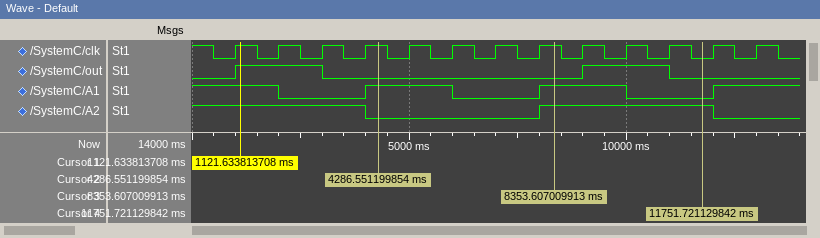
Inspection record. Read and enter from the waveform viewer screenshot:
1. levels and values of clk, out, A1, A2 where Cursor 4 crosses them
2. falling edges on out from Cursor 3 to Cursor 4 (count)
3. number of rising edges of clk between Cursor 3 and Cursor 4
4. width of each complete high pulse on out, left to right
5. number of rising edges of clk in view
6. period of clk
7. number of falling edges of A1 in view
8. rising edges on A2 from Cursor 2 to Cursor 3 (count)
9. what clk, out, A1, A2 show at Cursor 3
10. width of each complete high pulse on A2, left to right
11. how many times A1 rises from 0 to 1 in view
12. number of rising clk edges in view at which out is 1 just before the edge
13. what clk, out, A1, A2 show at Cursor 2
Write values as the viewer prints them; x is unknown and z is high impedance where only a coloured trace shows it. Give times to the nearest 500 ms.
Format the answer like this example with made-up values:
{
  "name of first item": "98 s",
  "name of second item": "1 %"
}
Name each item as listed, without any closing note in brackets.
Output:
{
  "levels and values of clk, out, A1, A2 where Cursor 4 crosses them": "clk=0, out=0, A1=0, A2=1",
  "falling edges on out from Cursor 3 to Cursor 4": "1",
  "number of rising edges of clk between Cursor 3 and Cursor 4": "3",
  "width of each complete high pulse on out, left to right": "2000 ms, 2000 ms",
  "number of rising edges of clk in view": "13",
  "period of clk": "1000 ms",
  "number of falling edges of A1 in view": "3",
  "rising edges on A2 from Cursor 2 to Cursor 3": "1",
  "what clk, out, A1, A2 show at Cursor 3": "clk=1, out=0, A1=1, A2=1",
  "width of each complete high pulse on A2, left to right": "4000 ms",
  "how many times A1 rises from 0 to 1 in view": "3",
  "number of rising clk edges in view at which out is 1 just before the edge": "4",
  "what clk, out, A1, A2 show at Cursor 2": "clk=1, out=0, A1=1, A2=0"
}
